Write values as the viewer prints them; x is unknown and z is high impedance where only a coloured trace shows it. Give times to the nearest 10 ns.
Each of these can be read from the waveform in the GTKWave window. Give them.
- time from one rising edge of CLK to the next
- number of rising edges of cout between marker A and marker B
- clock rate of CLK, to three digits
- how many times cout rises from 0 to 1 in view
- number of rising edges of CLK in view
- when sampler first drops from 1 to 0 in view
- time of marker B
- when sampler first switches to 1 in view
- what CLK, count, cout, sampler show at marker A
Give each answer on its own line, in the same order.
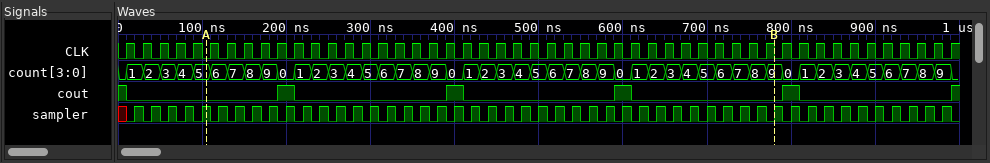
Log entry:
20 ns
3
50.0 MHz
5
50
30 ns
780 ns
20 ns
CLK=0, count=5, cout=0, sampler=1
